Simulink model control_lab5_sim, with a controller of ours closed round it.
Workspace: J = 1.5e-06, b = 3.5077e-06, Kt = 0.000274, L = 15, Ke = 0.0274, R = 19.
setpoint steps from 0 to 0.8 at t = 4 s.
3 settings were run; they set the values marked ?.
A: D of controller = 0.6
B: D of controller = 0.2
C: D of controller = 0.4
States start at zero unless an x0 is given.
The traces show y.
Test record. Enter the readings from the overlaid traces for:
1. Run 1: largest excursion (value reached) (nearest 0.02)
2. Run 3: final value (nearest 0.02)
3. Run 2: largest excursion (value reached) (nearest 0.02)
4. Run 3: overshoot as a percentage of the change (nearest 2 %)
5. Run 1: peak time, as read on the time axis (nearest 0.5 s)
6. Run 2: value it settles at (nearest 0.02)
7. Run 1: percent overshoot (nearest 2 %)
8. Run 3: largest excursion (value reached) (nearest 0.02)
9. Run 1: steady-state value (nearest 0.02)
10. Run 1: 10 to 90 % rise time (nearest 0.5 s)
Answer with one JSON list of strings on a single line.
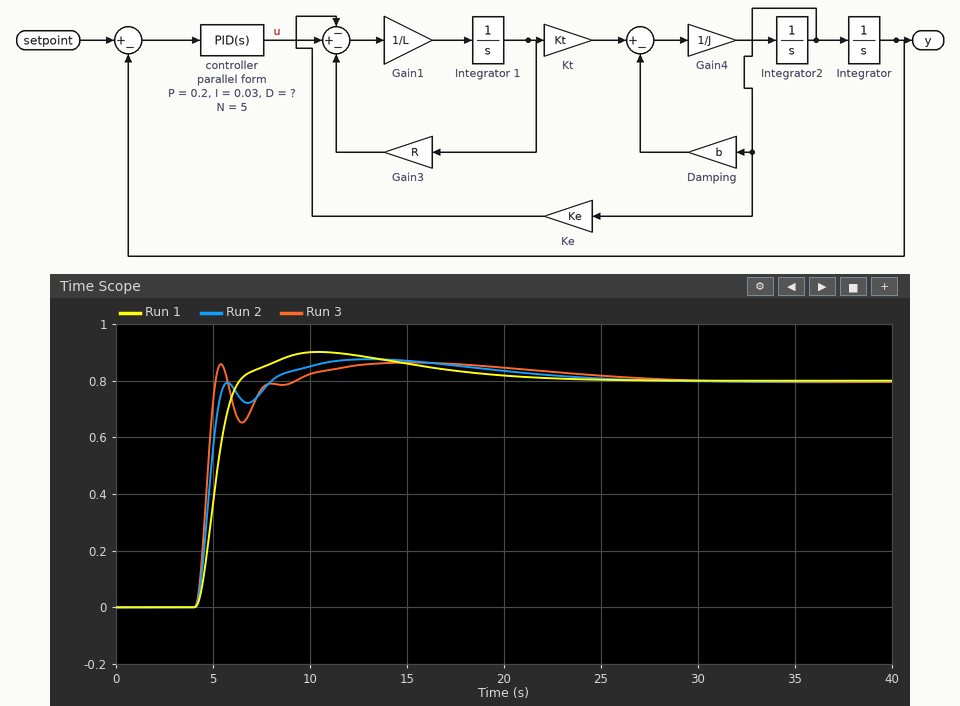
["0.90", "0.80", "0.88", "8 %", "10.5 s", "0.80", "12 %", "0.86", "0.80", "1.5 s"]
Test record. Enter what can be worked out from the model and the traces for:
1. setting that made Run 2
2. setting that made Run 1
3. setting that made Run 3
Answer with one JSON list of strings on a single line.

["C", "B", "A"]
